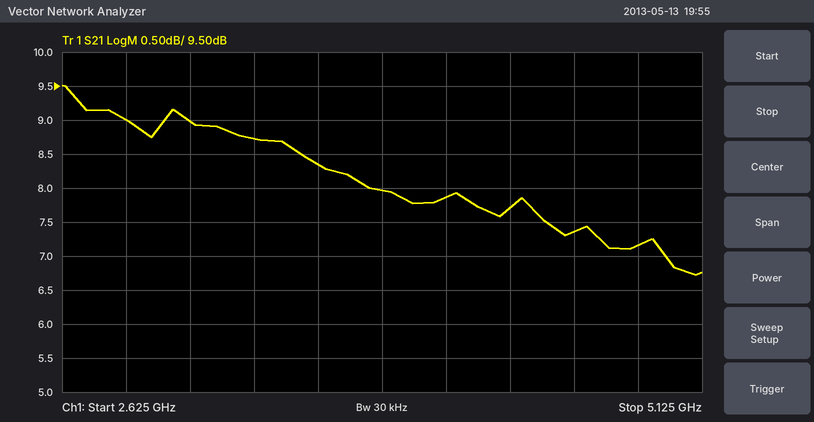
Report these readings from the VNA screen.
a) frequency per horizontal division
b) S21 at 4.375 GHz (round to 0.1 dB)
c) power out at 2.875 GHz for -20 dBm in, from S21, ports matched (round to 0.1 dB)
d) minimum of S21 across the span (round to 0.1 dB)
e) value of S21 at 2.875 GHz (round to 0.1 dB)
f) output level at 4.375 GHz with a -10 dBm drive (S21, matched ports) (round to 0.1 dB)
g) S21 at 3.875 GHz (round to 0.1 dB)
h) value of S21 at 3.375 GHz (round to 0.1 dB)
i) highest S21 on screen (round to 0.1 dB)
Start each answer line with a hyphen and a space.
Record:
- 250 MHz
- 7.7 dB
- -11.0 dBm
- 6.7 dB
- 9.0 dB
- -2.3 dBm
- 8.0 dB
- 8.7 dB
- 9.5 dB
